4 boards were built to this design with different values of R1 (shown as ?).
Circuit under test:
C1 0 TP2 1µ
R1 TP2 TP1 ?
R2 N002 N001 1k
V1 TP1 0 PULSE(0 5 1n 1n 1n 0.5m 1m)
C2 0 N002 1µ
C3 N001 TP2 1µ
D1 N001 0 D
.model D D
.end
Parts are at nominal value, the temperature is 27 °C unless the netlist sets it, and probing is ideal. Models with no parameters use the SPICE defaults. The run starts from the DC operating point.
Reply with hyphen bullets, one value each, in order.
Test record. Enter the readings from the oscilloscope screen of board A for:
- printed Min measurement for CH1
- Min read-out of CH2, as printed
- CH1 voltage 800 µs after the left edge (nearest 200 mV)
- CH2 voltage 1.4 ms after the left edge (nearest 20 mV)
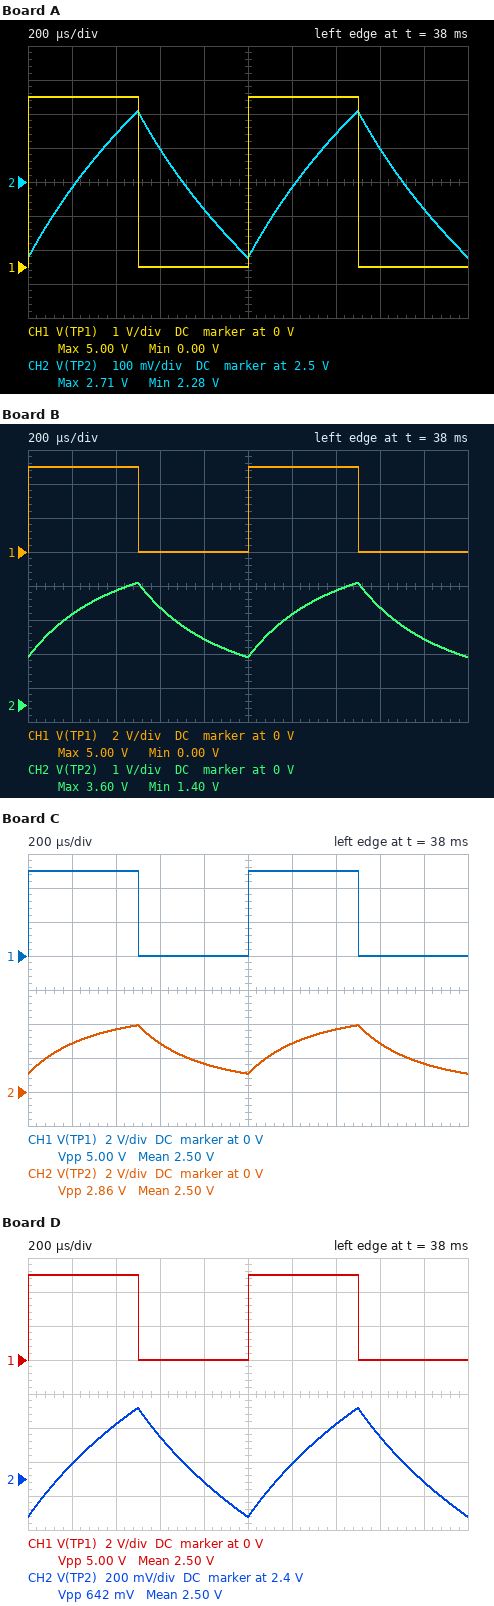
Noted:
- 0.00 V
- 2.28 V
- 0 V
- 2.64 V
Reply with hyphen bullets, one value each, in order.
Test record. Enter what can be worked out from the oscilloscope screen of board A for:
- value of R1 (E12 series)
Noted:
- 2.7 kΩ
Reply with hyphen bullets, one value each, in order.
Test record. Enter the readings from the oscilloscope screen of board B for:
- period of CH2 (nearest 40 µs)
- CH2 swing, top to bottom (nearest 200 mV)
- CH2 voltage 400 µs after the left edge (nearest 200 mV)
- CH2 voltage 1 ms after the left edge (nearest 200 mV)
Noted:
- 1.00 ms
- 2.2 V
- 3.4 V
- 1.4 V
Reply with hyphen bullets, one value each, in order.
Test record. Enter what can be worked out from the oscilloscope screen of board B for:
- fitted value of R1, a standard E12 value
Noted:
- 470 Ω
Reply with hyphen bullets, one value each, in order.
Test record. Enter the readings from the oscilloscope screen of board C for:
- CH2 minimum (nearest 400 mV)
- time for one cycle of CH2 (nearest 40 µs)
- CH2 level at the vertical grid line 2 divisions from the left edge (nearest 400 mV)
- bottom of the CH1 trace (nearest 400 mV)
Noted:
- 1.2 V
- 1.00 ms
- 3.6 V
- 0 V
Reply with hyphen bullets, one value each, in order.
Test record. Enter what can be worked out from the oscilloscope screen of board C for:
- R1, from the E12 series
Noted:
- 330 Ω
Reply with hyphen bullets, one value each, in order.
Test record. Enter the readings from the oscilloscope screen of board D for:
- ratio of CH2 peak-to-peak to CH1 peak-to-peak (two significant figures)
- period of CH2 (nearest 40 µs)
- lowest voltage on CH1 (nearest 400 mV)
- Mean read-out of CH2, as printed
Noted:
- 0.13
- 1.00 ms
- 0 V
- 2.50 V
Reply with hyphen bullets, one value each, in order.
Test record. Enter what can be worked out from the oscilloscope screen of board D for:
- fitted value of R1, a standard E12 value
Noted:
- 1.8 kΩ
